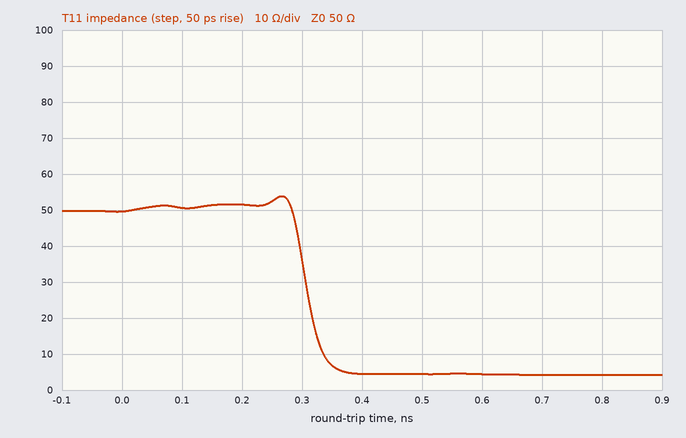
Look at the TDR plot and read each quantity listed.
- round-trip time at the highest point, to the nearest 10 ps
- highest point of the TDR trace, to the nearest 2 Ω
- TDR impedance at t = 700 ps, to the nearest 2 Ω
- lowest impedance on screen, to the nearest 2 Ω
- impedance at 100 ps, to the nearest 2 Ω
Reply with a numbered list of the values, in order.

1. 270 ps
2. 54 Ω
3. 4 Ω
4. 4 Ω
5. 50 Ω
